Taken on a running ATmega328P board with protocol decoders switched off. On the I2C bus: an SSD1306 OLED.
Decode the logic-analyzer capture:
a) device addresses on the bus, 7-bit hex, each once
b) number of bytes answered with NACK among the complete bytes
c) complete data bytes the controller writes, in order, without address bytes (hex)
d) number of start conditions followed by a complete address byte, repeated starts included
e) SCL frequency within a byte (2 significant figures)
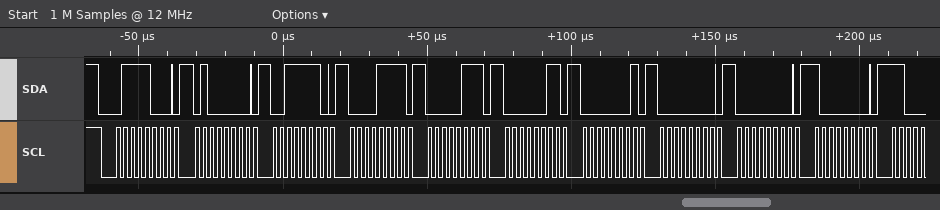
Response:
0x3C
0
40 3E 0F 07 03 01 00 00 80
1
400 kHz
